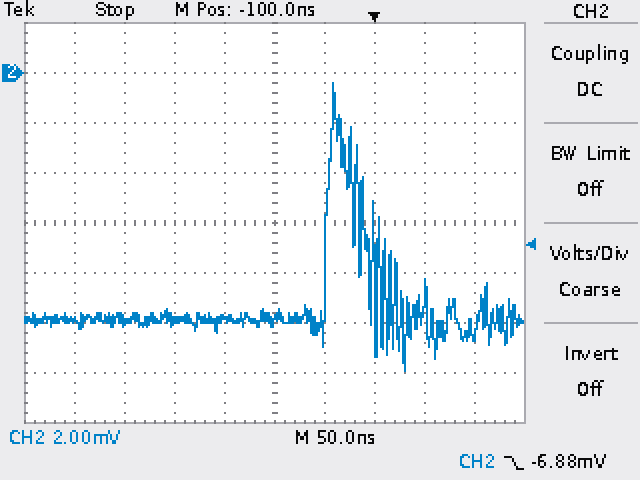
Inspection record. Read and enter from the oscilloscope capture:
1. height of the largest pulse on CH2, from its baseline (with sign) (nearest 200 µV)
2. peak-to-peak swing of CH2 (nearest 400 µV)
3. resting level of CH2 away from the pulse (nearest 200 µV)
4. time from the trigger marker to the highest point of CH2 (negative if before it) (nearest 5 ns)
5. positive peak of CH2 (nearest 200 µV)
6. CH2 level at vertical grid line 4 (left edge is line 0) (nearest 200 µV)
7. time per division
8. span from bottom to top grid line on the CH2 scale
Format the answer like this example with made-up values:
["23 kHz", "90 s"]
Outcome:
["+9.4 mV", "11.6 mV", "-9.8 mV", "-40 ns", "-400 µV", "-9.8 mV", "50 ns", "16 mV"]
